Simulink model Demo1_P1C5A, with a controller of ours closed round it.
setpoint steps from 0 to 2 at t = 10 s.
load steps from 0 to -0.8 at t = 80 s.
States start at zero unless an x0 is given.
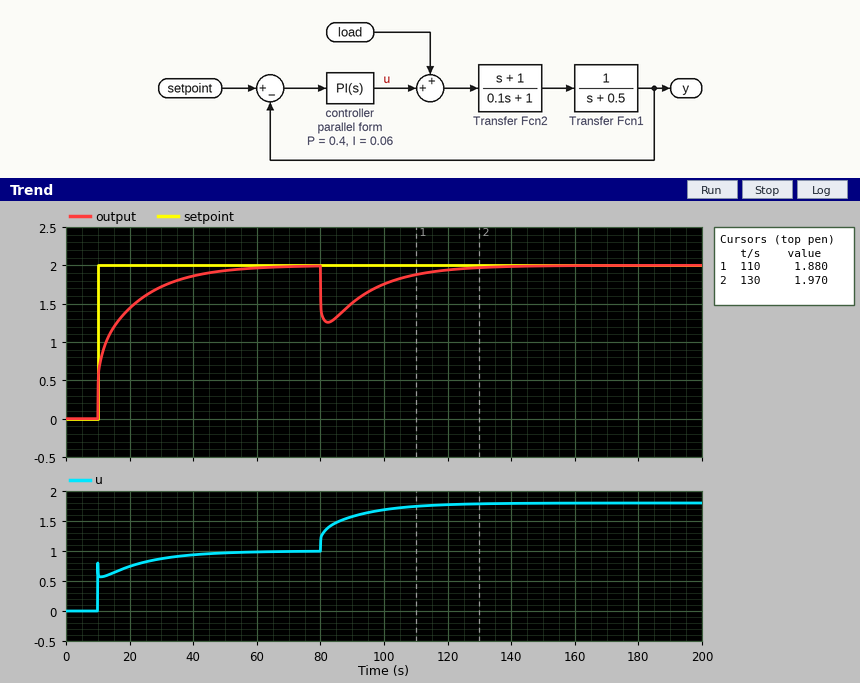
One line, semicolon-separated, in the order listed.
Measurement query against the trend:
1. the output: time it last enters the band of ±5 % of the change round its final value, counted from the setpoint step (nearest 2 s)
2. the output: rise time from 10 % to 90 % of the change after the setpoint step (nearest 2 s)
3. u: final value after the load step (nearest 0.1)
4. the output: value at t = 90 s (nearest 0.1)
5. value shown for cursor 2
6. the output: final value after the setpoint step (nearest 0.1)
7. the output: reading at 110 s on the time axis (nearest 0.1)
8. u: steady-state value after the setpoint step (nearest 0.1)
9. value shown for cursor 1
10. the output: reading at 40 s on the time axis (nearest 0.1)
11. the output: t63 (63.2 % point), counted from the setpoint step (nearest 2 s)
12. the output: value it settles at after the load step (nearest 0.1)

34 s; 24 s; 1.8; 1.5; 1.970; 2.0; 1.9; 1.0; 1.880; 1.9; 6 s; 2.0
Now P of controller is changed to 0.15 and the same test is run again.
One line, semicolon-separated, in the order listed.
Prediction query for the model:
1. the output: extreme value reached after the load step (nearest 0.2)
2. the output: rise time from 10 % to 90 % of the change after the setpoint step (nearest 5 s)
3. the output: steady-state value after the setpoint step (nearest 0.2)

1.0; 20 s; 2.0
